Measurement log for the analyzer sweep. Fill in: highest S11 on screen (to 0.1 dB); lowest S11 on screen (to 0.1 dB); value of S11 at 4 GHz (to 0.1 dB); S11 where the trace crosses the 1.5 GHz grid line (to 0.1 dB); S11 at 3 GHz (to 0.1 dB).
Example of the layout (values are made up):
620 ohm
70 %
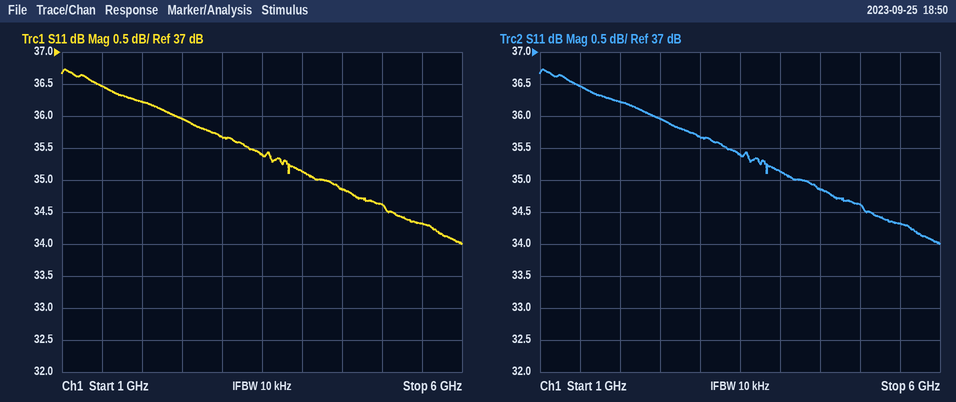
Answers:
36.7 dB
34.0 dB
35.1 dB
36.5 dB
35.7 dB
